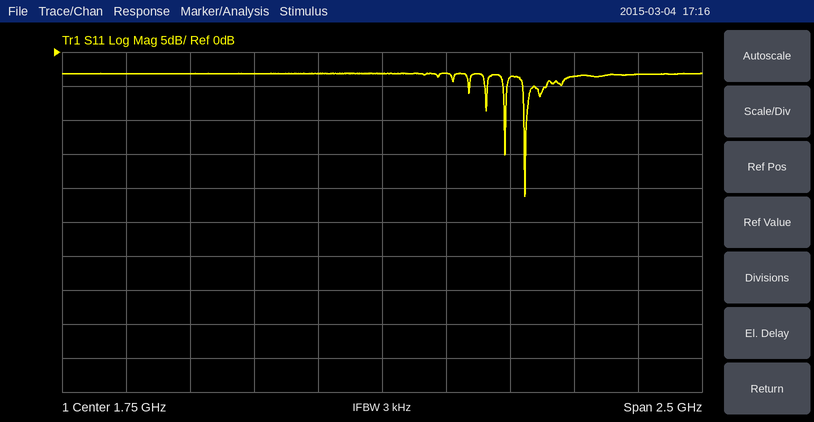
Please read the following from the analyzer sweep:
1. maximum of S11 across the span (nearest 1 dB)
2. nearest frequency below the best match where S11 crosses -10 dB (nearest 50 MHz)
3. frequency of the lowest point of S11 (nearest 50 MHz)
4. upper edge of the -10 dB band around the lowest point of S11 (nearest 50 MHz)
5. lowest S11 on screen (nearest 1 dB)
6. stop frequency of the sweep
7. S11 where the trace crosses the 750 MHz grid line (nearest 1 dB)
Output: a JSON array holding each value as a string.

["-3 dB", "2.30 GHz", "2.30 GHz", "2.30 GHz", "-21 dB", "3 GHz", "-3 dB"]
